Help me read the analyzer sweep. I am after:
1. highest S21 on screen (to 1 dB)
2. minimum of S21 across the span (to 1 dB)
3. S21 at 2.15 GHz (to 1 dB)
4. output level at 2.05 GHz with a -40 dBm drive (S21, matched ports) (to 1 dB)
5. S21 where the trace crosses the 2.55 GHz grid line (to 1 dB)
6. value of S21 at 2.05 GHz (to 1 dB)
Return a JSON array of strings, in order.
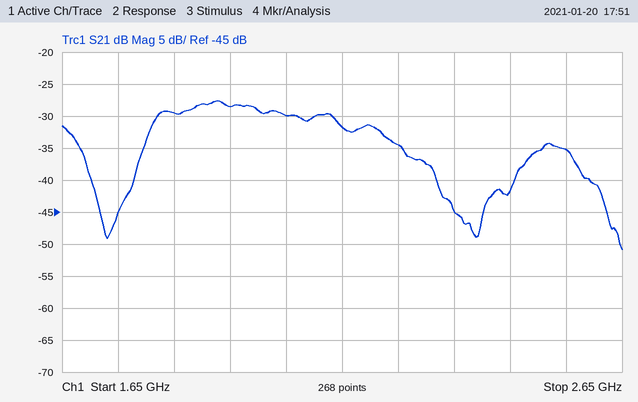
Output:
["-28 dB", "-51 dB", "-32 dB", "-70 dBm", "-35 dB", "-30 dB"]
